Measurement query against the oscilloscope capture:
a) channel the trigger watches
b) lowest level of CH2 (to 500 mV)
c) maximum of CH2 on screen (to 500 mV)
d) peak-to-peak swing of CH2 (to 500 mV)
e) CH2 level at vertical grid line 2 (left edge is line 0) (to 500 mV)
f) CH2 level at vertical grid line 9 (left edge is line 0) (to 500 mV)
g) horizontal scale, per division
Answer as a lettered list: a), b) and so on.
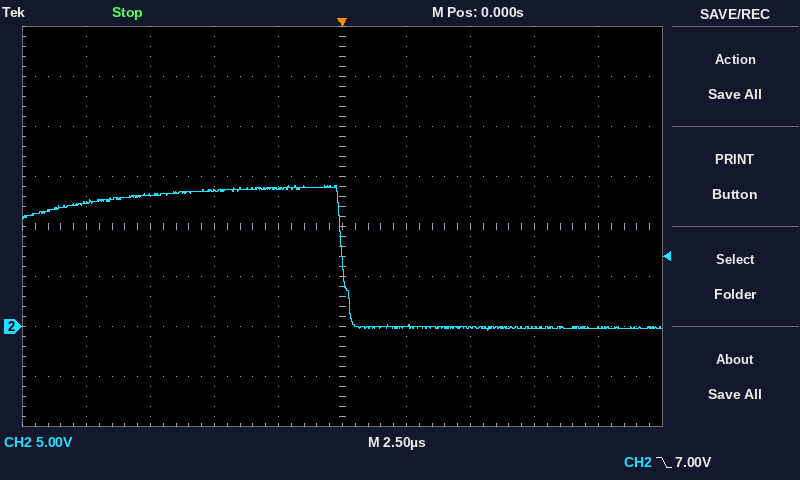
a) CH2
b) -500 mV
c) 14.0 V
d) 14.5 V
e) 13.0 V
f) 0.0 V
g) 2.5 µs
